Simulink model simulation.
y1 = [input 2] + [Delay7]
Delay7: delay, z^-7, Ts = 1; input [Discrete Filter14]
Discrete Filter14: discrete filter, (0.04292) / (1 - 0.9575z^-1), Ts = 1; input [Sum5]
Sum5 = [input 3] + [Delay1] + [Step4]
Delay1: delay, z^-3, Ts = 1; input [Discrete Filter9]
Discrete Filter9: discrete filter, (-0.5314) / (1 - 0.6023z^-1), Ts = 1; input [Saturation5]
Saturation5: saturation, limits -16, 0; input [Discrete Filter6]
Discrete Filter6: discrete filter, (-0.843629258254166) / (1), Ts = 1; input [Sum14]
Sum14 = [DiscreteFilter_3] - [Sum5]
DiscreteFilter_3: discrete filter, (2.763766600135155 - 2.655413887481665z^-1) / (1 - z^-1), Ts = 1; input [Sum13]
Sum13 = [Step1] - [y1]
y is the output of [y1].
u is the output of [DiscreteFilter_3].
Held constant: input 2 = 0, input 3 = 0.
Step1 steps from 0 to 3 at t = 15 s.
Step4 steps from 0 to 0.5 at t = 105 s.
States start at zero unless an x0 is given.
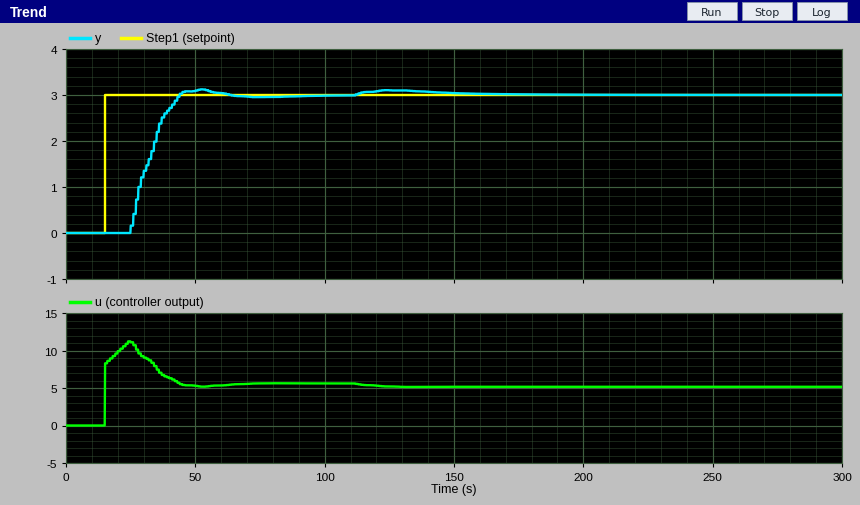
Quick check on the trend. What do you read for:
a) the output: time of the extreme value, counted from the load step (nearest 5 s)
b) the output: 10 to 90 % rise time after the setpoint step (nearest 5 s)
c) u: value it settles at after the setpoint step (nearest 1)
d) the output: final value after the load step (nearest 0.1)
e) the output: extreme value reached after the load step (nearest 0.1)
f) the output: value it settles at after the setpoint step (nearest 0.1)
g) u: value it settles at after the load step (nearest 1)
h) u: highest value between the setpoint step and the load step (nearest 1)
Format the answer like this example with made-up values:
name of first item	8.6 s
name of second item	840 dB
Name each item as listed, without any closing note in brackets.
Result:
the output: time of the extreme value, counted from the load step	20 s
the output: 10 to 90 % rise time after the setpoint step	15 s
u: value it settles at after the setpoint step	6
the output: final value after the load step	3.0
the output: extreme value reached after the load step	3.1
the output: value it settles at after the setpoint step	3.0
u: value it settles at after the load step	5
u: highest value between the setpoint step and the load step	11
